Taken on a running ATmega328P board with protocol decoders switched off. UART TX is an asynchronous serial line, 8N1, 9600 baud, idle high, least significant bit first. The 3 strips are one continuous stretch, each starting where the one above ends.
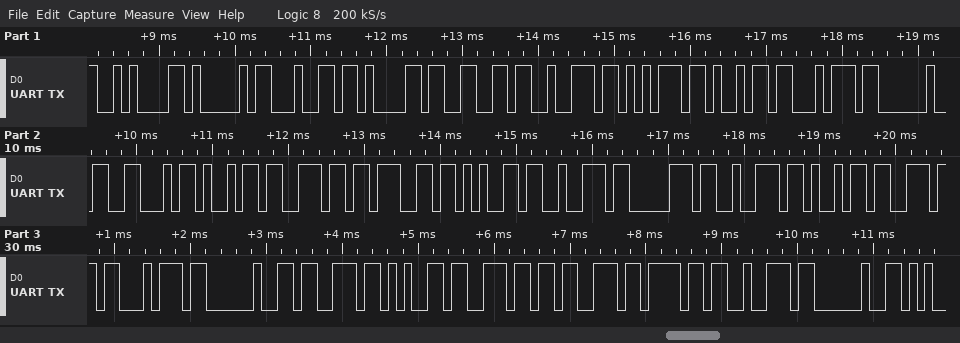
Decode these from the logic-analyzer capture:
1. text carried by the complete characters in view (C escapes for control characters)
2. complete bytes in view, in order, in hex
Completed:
"\nAdafruit Fingerprint sensor "
0A 41 64 61 66 72 75 69 74 20 46 69 6E 67 65 72 70 72 69 6E 74 20 73 65 6E 73 6F 72 20
